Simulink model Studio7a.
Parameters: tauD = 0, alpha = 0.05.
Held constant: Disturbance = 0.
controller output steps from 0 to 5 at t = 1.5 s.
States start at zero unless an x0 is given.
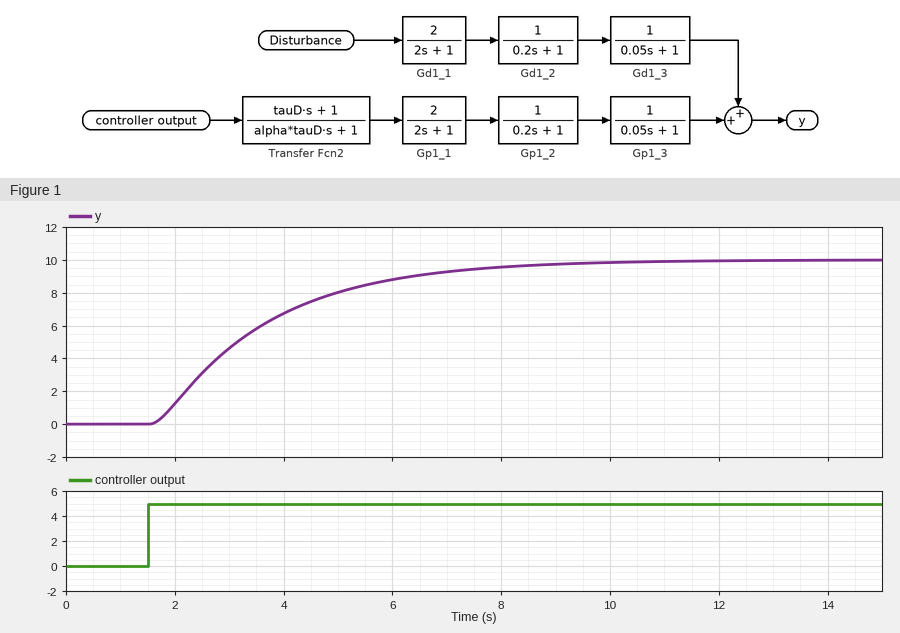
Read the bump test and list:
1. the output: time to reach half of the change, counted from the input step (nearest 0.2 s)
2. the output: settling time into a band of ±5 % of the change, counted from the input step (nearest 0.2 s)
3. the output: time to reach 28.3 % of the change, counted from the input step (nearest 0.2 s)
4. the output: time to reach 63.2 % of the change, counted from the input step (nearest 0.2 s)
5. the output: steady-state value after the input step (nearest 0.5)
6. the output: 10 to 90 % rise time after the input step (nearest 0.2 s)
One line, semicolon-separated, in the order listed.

1.6 s; 6.2 s; 1.0 s; 2.2 s; 10.0; 4.4 s
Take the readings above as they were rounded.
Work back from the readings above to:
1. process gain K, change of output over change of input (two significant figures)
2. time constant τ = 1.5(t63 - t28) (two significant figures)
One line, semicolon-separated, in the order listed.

2.0; 1.8 s
